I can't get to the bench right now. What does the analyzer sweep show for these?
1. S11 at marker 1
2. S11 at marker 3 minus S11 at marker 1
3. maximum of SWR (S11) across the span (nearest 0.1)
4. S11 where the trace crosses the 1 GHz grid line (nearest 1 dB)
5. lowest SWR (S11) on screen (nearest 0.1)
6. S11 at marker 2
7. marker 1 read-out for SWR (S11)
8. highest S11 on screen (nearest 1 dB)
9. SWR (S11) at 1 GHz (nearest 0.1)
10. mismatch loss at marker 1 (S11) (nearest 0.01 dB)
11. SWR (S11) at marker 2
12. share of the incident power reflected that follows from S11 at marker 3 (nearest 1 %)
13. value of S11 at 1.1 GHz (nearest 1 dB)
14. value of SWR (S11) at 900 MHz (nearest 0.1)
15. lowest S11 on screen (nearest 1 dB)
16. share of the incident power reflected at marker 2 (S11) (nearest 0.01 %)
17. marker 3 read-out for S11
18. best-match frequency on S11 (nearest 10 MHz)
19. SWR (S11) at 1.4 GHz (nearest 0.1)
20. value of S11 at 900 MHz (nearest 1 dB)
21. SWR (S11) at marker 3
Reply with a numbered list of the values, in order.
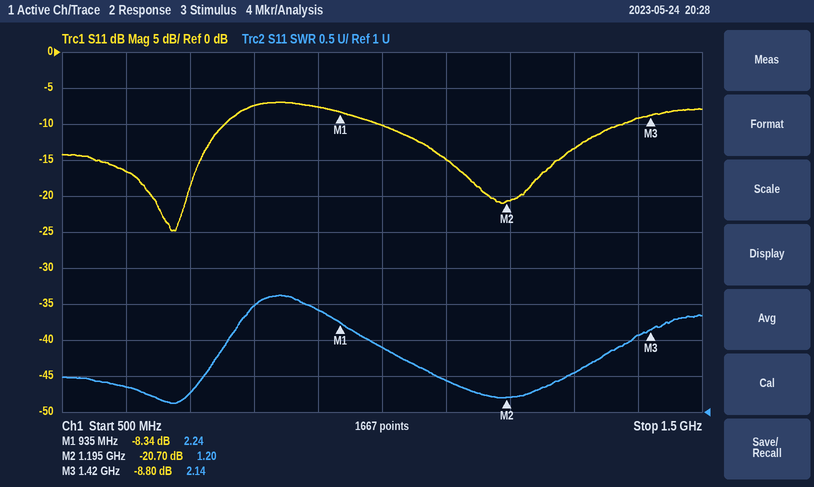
1. -8.34 dB
2. -0.46 dB
3. 2.6
4. -10 dB
5. 1.1
6. -20.70 dB
7. 2.24
8. -7 dB
9. 1.9
10. 0.69 dB
11. 1.20
12. 13 %
13. -15 dB
14. 2.4
15. -25 dB
16. 0.85 %
17. -8.80 dB
18. 670 MHz
19. 2.1
20. -8 dB
21. 2.14
